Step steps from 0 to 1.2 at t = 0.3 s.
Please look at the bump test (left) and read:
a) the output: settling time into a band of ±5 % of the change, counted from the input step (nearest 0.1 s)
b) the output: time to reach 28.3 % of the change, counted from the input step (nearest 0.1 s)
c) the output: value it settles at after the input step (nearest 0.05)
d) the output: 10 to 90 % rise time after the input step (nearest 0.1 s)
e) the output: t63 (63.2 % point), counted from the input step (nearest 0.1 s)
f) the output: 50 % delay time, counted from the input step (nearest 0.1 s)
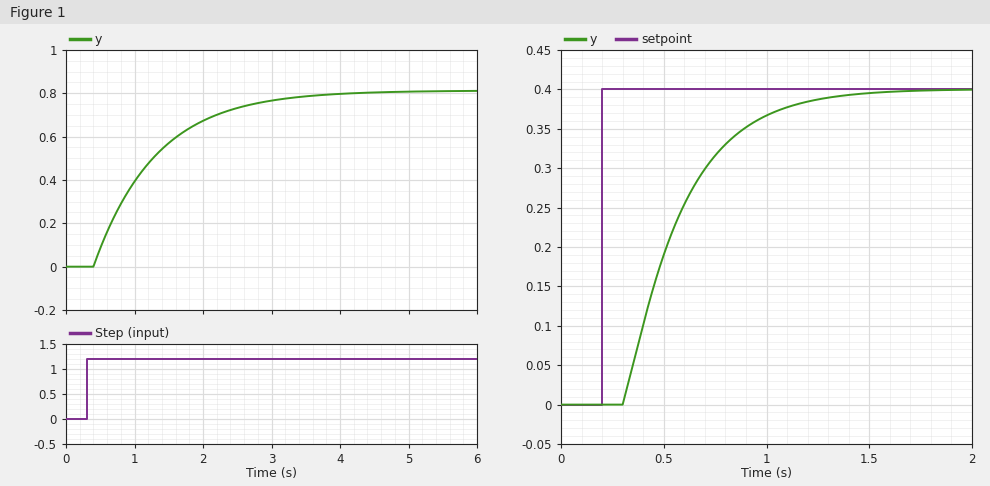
2.8 s
0.4 s
0.80
2.0 s
1.0 s
0.7 s
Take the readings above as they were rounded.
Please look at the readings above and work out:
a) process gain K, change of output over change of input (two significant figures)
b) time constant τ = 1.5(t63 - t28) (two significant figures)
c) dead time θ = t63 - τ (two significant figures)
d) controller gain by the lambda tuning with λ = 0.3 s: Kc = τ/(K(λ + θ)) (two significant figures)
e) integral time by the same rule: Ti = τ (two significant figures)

0.67
0.90 s
0.10 s
3.4
0.90 s
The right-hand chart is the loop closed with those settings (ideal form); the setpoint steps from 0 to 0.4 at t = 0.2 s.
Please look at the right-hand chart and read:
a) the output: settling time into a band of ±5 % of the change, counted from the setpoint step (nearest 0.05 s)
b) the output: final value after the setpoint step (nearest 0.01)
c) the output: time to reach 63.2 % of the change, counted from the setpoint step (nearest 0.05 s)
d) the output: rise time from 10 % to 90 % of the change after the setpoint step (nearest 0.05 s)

0.95 s
0.40
0.40 s
0.60 s
